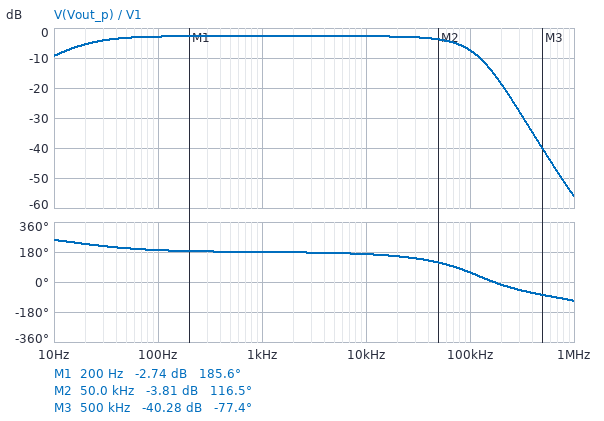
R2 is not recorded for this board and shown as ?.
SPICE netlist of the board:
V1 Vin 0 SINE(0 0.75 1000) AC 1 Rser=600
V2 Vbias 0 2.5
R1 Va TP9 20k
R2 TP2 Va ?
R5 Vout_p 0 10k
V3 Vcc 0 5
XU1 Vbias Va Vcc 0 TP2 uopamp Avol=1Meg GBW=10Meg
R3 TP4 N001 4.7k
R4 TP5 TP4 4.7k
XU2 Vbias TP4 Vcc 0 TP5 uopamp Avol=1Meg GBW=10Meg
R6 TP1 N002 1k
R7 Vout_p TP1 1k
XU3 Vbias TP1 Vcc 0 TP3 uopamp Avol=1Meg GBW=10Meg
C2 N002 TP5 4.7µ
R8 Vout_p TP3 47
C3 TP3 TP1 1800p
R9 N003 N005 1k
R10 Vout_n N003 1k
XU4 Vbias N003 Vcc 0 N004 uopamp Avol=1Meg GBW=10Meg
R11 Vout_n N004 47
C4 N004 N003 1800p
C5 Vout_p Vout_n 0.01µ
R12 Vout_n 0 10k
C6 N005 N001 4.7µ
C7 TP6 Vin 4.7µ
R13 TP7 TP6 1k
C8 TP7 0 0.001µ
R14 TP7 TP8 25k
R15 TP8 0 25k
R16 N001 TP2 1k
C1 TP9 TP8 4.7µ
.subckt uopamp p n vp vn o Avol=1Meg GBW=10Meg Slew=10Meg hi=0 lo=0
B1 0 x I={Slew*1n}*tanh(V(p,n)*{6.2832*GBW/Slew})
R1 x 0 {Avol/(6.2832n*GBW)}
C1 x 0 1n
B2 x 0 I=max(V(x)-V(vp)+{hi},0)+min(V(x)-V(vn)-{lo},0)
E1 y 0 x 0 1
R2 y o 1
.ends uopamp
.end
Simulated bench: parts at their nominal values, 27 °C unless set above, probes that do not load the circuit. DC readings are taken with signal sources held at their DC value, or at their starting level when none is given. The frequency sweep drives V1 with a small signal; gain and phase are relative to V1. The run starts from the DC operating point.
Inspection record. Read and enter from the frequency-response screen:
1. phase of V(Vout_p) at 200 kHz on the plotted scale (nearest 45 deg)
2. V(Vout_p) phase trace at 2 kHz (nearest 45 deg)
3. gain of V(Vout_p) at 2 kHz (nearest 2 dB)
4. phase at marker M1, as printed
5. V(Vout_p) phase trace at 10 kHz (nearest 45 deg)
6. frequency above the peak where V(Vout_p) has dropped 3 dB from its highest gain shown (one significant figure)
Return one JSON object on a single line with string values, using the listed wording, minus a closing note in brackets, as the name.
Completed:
{"phase of V(Vout_p) at 200 kHz on the plotted scale": "0 deg", "V(Vout_p) phase trace at 2 kHz": "180 deg", "gain of V(Vout_p) at 2 kHz": "-2 dB", "phase at marker M1, as printed": "185.6 deg", "V(Vout_p) phase trace at 10 kHz": "180 deg", "frequency above the peak where V(Vout_p) has dropped 3 dB from its highest gain shown": "80 kHz"}
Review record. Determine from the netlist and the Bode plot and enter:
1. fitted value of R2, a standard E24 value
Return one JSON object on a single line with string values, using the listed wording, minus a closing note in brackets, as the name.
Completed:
{"fitted value of R2, a standard E24 value": "110 kΩ"}
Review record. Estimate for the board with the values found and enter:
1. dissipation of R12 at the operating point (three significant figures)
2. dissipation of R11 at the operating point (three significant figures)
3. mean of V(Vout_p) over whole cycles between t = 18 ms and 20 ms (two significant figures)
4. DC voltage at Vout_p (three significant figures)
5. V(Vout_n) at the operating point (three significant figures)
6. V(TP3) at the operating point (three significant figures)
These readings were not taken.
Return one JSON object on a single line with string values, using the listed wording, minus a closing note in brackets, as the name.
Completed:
{"dissipation of R12 at the operating point": "625 µW", "dissipation of R11 at the operating point": "2.94 µW", "mean of V(Vout_p) over whole cycles between t = 18 ms and 20 ms": "2.5 V", "DC voltage at Vout_p": "2.50 V", "V(Vout_n) at the operating point": "2.50 V", "V(TP3) at the operating point": "2.51 V"}
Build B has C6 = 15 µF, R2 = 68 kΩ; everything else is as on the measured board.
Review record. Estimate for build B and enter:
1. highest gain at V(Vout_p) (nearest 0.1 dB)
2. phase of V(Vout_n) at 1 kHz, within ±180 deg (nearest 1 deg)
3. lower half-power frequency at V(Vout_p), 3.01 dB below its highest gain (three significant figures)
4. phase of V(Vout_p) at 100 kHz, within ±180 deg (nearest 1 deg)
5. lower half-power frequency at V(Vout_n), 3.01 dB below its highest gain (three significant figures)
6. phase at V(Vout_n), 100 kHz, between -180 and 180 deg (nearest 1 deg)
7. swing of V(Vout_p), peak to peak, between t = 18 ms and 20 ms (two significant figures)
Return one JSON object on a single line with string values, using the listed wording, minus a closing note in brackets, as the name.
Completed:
{"highest gain at V(Vout_p)": "-6.9 dB", "phase of V(Vout_n) at 1 kHz, within ±180 deg": "-1 deg", "lower half-power frequency at V(Vout_p), 3.01 dB below its highest gain": "31.6 Hz", "phase of V(Vout_p) at 100 kHz, within ±180 deg": "58 deg", "lower half-power frequency at V(Vout_n), 3.01 dB below its highest gain": "6.19 Hz", "phase at V(Vout_n), 100 kHz, between -180 and 180 deg": "-121 deg", "swing of V(Vout_p), peak to peak, between t = 18 ms and 20 ms": "680 mV"}
